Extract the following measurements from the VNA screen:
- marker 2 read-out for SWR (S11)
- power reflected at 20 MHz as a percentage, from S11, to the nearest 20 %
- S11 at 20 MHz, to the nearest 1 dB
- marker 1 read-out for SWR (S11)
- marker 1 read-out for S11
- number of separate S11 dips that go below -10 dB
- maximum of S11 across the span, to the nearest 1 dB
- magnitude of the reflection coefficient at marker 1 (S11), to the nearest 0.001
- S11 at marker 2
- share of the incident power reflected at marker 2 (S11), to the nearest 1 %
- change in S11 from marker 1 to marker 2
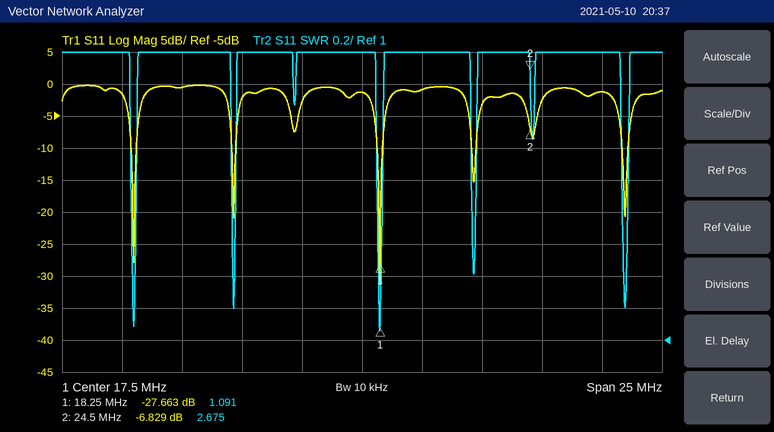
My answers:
2.675
80 %
-1 dB
1.091
-27.663 dB
5
0 dB
0.041
-6.829 dB
21 %
20.834 dB
